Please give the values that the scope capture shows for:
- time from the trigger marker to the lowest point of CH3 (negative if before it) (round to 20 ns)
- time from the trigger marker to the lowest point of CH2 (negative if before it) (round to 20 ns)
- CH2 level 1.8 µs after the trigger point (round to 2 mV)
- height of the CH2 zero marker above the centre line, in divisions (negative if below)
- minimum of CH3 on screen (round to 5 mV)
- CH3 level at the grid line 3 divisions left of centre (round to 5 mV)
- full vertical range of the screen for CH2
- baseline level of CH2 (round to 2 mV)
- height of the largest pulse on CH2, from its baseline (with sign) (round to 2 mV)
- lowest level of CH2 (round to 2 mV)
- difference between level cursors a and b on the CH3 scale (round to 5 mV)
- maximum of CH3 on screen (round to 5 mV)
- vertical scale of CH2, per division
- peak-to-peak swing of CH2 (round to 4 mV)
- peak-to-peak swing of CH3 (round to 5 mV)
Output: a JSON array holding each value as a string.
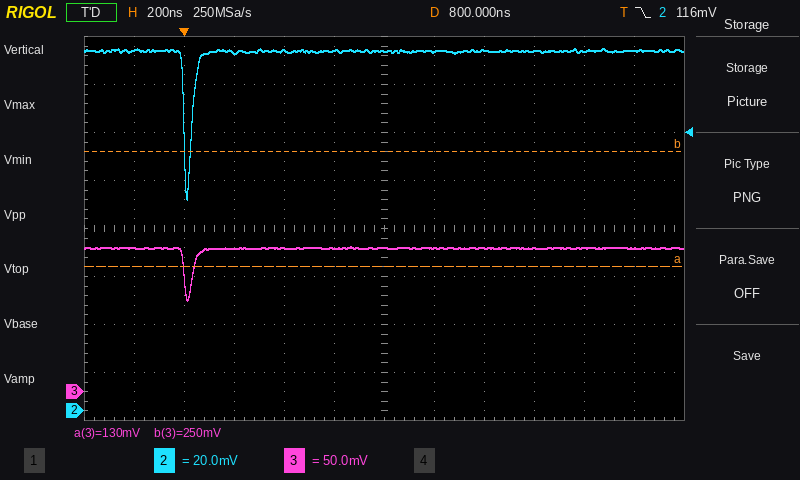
["+20 ns", "+20 ns", "150 mV", "-3.8 div", "95 mV", "150 mV", "160 mV", "150 mV", "-62 mV", "88 mV", "120 mV", "150 mV", "20 mV", "64 mV", "55 mV"]
